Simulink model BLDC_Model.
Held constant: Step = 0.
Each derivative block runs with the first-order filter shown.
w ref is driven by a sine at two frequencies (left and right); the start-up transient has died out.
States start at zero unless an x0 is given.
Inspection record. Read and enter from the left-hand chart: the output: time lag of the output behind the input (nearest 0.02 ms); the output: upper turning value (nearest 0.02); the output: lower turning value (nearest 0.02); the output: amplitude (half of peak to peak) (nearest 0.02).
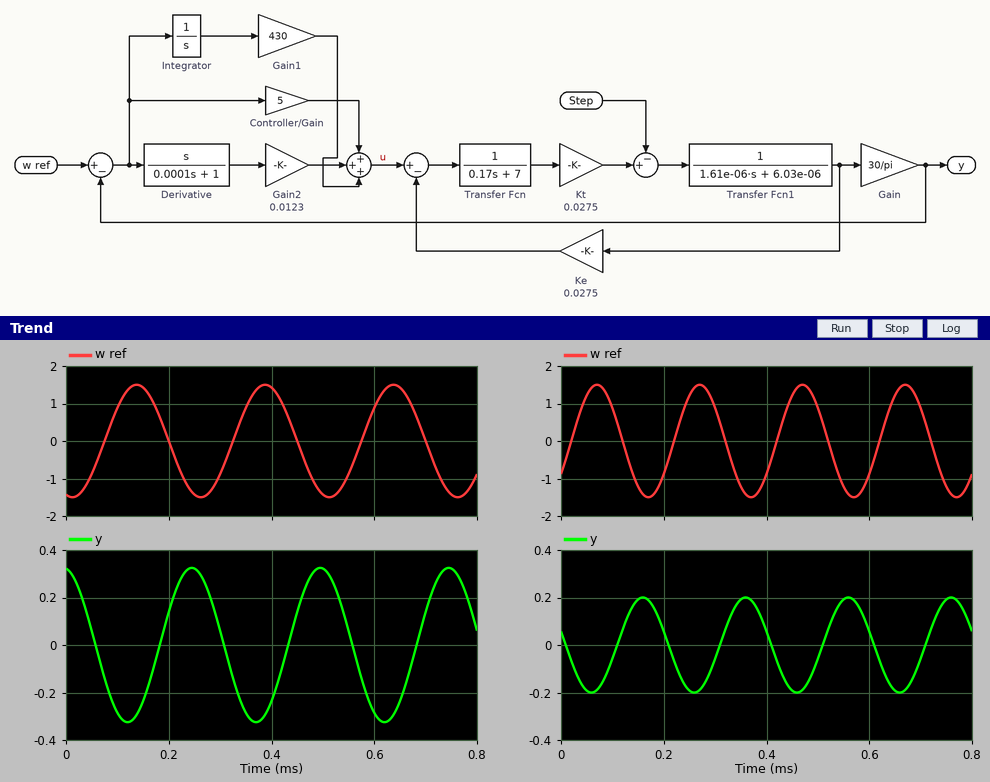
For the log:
0.10 ms
0.32
-0.32
0.32
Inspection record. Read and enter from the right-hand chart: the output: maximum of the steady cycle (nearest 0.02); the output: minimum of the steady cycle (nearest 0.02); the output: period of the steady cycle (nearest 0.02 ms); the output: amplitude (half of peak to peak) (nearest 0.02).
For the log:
0.20
-0.20
0.20 ms
0.20
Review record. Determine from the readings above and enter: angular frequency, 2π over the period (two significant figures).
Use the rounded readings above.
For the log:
31 rad/ms
